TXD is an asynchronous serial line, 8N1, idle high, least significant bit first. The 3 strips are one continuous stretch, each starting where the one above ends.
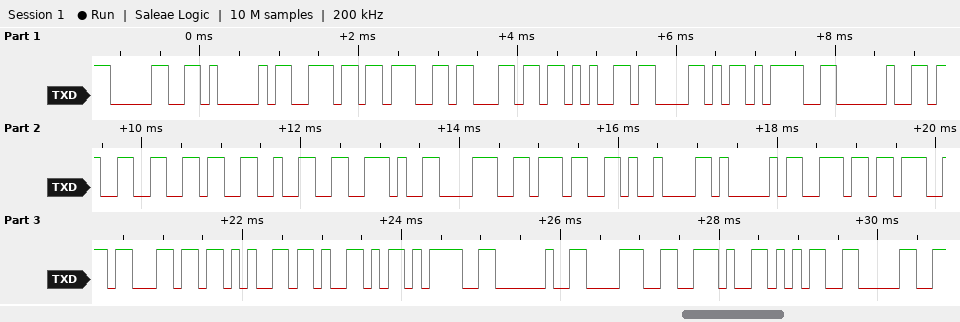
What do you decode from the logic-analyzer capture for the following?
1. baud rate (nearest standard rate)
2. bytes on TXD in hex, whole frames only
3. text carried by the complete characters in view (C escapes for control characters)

9600 baud
30 41 6E 67 6C 65 58 3D 20 33 36 32 2E 38 37 09 41 6E 67 6C 65 59 3D 20 38 2E 35 30
"0AngleX= 362.87\tAngleY= 8.50"
